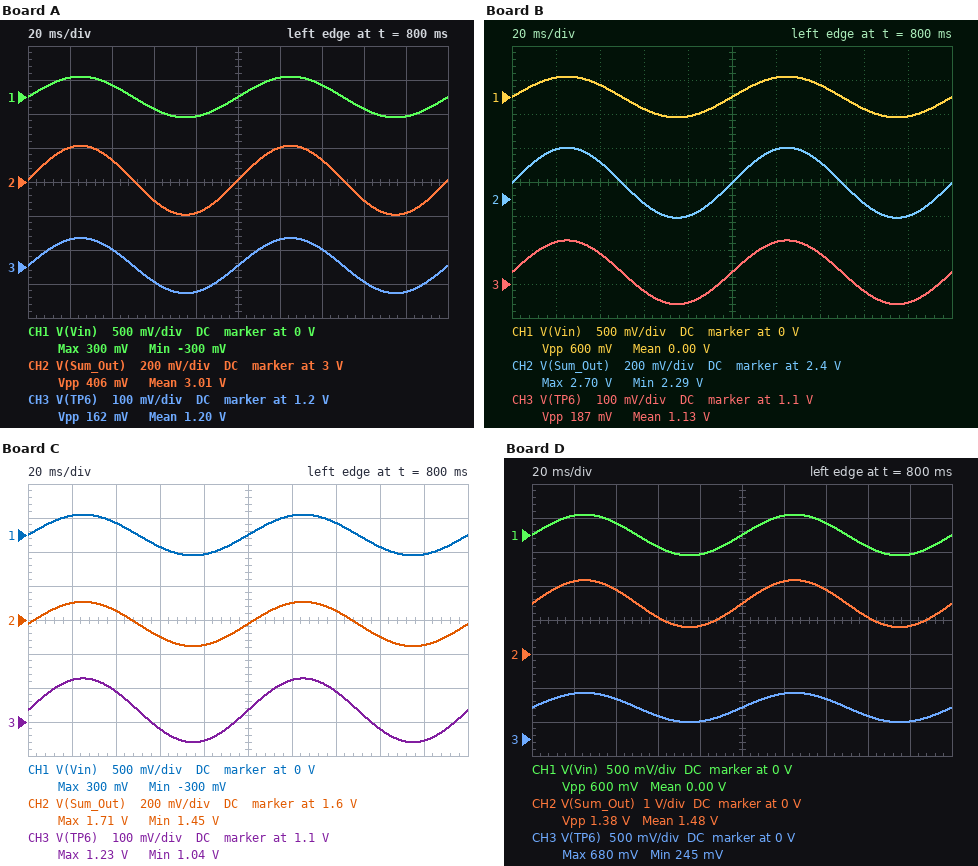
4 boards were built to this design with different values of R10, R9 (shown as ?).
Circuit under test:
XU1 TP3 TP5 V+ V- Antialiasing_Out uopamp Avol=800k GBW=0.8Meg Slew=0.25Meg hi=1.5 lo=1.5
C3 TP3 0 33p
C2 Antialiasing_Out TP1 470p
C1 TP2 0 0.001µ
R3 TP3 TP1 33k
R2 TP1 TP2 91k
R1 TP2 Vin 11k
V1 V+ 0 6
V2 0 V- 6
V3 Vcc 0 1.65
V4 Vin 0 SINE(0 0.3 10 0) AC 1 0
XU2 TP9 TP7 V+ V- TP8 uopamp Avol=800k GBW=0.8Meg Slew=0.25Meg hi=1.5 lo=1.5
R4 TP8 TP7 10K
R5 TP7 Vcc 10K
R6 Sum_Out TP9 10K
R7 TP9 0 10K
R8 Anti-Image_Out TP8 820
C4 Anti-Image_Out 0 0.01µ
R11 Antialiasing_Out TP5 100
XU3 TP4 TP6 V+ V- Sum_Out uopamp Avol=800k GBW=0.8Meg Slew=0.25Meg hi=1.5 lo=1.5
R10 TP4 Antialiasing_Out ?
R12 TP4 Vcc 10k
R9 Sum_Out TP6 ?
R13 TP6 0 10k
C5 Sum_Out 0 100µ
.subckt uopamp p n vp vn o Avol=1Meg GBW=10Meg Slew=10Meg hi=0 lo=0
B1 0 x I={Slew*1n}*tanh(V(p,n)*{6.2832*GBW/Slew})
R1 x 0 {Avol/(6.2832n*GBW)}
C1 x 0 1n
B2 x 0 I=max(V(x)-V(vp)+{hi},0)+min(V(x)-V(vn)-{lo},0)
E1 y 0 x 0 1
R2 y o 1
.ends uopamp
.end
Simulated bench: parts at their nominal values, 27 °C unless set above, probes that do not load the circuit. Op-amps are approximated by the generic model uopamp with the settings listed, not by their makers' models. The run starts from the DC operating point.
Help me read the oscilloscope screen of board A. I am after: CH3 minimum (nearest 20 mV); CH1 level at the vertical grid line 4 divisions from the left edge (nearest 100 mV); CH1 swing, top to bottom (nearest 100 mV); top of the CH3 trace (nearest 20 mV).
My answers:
1.12 V
-300 mV
600 mV
1.28 V
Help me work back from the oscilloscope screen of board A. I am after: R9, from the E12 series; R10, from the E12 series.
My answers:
15 kΩ
27 kΩ
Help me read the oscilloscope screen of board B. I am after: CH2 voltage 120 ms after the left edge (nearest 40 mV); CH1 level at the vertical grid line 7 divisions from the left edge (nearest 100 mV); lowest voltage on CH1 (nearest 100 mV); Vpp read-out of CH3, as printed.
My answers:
2.68 V
200 mV
-300 mV
187 mV
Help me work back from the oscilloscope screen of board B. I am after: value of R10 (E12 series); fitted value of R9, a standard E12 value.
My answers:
22 kΩ
12 kΩ
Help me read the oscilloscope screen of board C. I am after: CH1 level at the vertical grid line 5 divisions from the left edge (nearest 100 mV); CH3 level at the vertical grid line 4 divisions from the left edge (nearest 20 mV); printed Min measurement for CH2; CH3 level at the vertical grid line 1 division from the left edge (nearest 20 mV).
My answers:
0 V
1.04 V
1.45 V
1.22 V
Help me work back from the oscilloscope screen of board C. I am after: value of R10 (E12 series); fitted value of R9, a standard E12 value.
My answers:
22 kΩ
3.9 kΩ
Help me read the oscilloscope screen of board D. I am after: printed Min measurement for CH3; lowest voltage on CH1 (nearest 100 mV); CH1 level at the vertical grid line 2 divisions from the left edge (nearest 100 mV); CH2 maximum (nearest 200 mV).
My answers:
245 mV
-300 mV
200 mV
2.2 V
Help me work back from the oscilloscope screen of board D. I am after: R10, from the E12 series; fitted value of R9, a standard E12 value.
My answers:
3.9 kΩ
22 kΩ
